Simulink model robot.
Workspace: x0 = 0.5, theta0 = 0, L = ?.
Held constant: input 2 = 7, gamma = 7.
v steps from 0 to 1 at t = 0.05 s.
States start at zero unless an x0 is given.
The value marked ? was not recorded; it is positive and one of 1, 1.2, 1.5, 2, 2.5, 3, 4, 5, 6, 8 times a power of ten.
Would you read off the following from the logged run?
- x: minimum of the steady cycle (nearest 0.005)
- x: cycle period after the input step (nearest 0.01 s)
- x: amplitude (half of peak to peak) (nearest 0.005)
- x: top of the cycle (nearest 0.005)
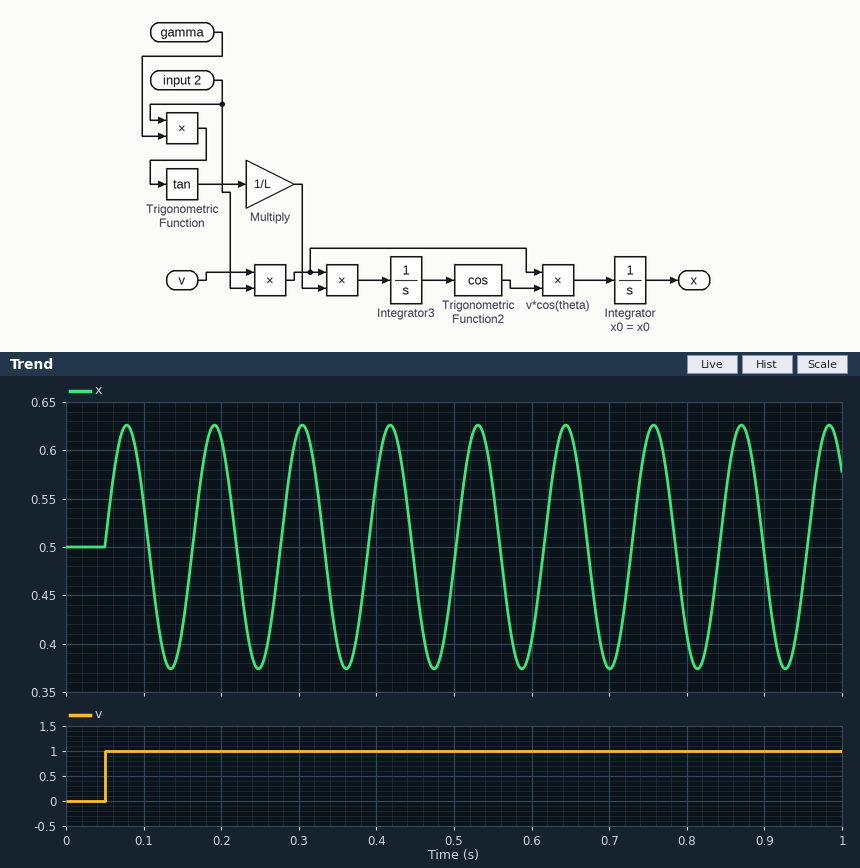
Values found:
0.375
0.11 s
0.125
0.625
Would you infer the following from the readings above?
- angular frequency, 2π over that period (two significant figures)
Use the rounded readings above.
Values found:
57 rad/s
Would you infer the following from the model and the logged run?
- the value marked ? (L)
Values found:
0.4
